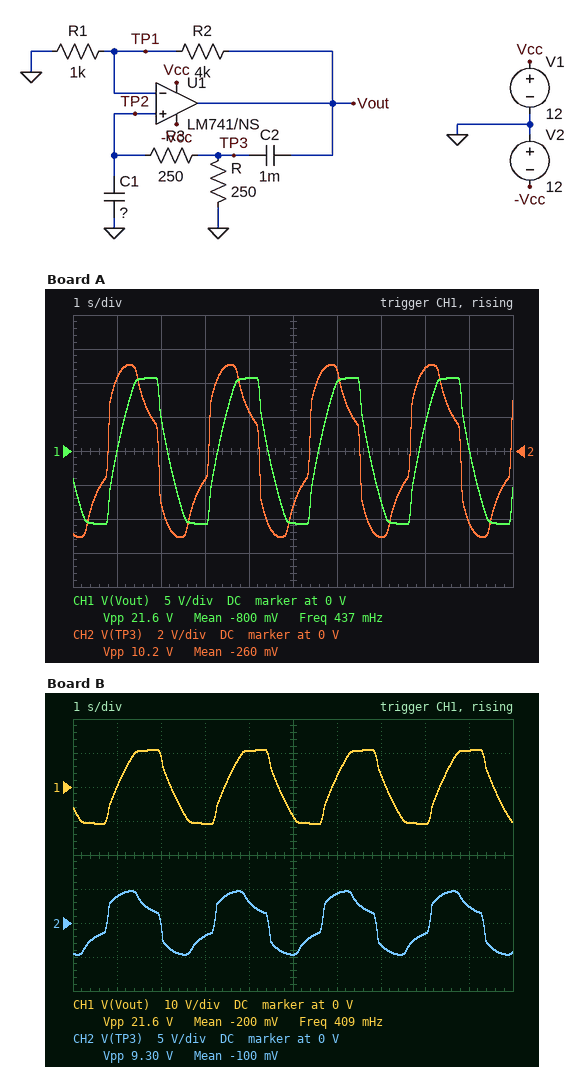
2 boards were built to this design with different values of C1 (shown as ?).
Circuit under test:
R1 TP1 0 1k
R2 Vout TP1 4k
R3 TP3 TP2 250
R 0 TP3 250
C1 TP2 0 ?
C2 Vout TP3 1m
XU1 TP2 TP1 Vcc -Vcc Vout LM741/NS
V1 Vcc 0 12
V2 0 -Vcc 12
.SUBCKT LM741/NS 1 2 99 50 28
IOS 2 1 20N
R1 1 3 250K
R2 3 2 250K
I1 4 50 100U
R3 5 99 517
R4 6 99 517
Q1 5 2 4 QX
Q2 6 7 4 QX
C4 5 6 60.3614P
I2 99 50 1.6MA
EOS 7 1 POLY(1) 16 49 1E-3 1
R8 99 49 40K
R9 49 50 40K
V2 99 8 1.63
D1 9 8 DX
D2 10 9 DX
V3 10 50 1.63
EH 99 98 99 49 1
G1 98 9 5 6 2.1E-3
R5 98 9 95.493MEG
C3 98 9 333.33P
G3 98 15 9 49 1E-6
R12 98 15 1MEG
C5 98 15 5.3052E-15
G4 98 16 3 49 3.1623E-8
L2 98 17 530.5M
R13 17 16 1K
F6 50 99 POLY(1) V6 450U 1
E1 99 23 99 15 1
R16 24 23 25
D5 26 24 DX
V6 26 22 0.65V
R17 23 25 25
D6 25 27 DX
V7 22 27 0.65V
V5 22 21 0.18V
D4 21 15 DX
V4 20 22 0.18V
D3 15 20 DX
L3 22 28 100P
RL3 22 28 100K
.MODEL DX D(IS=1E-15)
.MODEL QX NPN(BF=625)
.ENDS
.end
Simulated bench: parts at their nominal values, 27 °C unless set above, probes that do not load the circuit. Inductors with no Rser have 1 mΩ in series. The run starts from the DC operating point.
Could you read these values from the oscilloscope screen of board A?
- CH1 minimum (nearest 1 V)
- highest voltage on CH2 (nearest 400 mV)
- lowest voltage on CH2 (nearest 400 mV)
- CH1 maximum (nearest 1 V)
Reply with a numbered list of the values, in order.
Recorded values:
1. -11 V
2. 5.2 V
3. -5.2 V
4. 11 V
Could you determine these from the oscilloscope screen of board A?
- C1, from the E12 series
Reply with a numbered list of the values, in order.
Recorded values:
1. 560 µF
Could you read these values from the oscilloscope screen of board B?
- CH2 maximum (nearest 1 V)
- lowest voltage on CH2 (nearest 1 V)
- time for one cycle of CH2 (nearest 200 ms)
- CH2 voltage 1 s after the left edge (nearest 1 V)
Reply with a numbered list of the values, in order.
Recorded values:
1. 5 V
2. -5 V
3. 2.4 s
4. 4 V
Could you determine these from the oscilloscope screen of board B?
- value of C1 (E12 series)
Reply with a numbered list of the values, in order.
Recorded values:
1. 820 µF
